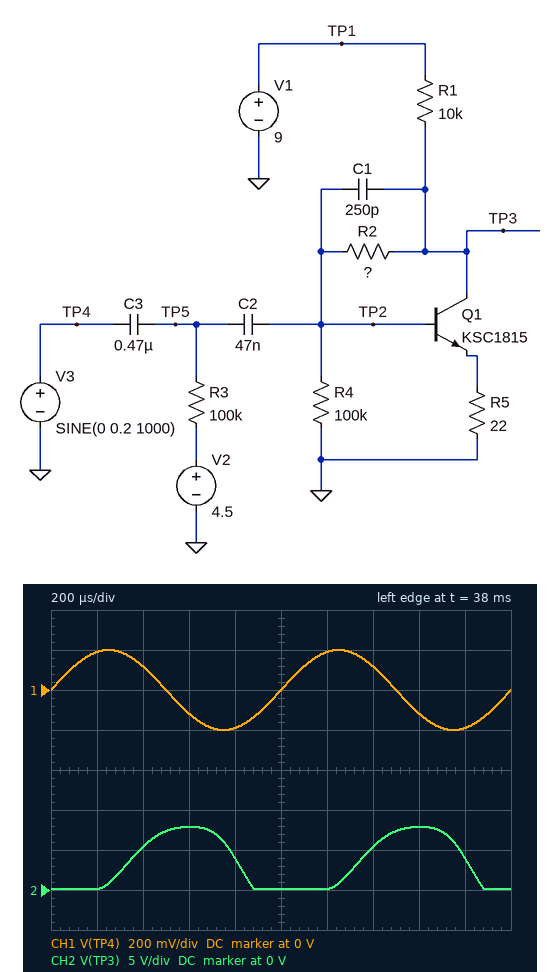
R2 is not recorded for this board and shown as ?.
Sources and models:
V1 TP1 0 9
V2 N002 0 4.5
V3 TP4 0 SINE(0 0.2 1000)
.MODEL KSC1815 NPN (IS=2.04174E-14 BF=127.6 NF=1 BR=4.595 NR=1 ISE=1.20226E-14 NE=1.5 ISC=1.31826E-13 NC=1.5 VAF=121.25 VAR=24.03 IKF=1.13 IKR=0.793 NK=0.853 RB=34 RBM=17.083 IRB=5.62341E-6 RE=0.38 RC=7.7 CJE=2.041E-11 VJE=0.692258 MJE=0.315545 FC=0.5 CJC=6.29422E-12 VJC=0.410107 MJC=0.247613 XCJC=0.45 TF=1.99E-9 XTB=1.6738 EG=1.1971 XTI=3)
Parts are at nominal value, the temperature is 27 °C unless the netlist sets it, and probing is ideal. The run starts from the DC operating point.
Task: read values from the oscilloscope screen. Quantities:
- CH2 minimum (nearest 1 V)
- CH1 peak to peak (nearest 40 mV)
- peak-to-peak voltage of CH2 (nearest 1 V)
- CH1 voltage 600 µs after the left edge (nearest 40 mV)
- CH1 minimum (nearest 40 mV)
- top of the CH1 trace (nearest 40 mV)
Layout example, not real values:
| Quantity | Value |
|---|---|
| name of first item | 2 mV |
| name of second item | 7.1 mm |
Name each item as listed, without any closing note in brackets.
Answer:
| Quantity | Value |
|---|---|
| CH2 minimum | 0 V |
| CH1 peak to peak | 400 mV |
| peak-to-peak voltage of CH2 | 8 V |
| CH1 voltage 600 µs after the left edge | -120 mV |
| CH1 minimum | -200 mV |
| top of the CH1 trace | 200 mV |
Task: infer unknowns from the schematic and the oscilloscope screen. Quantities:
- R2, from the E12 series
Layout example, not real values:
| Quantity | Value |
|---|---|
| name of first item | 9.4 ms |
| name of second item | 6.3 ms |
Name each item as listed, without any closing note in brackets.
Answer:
| Quantity | Value |
|---|---|
| R2, from the E12 series | 150 kΩ |
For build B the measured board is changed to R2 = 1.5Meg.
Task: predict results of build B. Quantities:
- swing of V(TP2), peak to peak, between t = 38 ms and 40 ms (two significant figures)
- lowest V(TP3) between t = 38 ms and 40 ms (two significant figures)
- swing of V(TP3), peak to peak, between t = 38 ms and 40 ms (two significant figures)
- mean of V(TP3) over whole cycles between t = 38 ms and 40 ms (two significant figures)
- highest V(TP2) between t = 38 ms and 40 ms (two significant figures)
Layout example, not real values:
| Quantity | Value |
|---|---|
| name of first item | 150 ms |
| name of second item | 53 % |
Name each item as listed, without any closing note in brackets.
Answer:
| Quantity | Value |
|---|---|
| swing of V(TP2), peak to peak, between t = 38 ms and 40 ms | 370 mV |
| lowest V(TP3) between t = 38 ms and 40 ms | 4.8 V |
| swing of V(TP3), peak to peak, between t = 38 ms and 40 ms | 4.2 V |
| mean of V(TP3) over whole cycles between t = 38 ms and 40 ms | 8.1 V |
| highest V(TP2) between t = 38 ms and 40 ms | 620 mV |
